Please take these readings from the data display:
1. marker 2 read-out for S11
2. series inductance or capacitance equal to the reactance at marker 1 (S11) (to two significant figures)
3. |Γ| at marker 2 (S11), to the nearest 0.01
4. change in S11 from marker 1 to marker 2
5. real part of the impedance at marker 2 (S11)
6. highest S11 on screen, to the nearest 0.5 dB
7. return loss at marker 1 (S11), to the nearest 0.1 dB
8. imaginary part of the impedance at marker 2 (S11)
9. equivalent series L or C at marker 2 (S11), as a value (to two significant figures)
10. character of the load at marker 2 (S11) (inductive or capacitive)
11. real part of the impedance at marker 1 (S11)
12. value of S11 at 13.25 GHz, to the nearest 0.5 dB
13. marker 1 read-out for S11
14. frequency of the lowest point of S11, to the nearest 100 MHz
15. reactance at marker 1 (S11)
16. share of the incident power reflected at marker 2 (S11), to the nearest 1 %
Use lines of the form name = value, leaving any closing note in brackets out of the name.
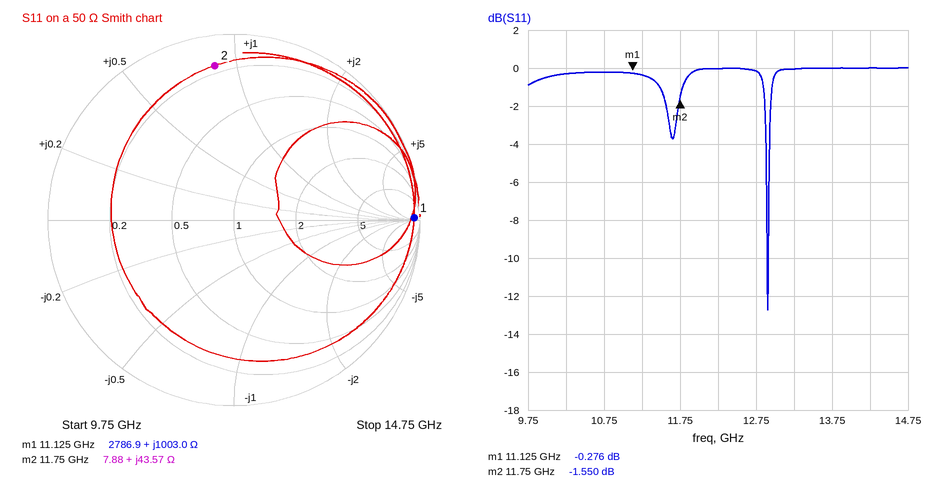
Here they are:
marker 2 read-out for S11 = -1.550 dB
series inductance or capacitance equal to the reactance at marker 1 (S11) = 14 nH
|Γ| at marker 2 (S11), to the nearest 0.01 = 0.84
change in S11 from marker 1 to marker 2 = -1.274 dB
real part of the impedance at marker 2 = 7.88 Ω
highest S11 on screen, to the nearest 0.5 dB = 0.0 dB
return loss at marker 1 (S11), to the nearest 0.1 dB = 0.3 dB
imaginary part of the impedance at marker 2 = +43.57 Ω
equivalent series L or C at marker 2 (S11), as a value = 590 pH
character of the load at marker 2 (S11) = inductive
real part of the impedance at marker 1 = 2786.9 Ω
value of S11 at 13.25 GHz, to the nearest 0.5 dB = 0.0 dB
marker 1 read-out for S11 = -0.276 dB
frequency of the lowest point of S11, to the nearest 100 MHz = 12.9 GHz
reactance at marker 1 = +1003.0 Ω
share of the incident power reflected at marker 2 (S11), to the nearest 1 % = 70 %
